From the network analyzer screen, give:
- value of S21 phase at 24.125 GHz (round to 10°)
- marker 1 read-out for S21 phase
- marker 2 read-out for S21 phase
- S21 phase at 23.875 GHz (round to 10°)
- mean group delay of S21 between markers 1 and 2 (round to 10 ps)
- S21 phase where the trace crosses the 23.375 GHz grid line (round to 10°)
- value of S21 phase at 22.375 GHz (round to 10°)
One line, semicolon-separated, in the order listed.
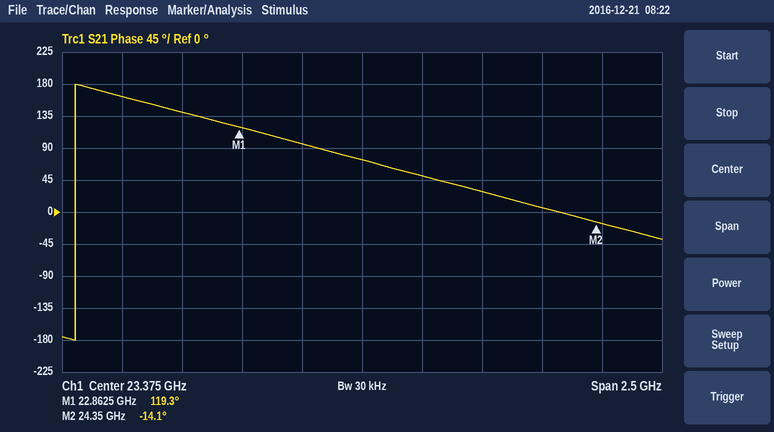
10°; 119.3°; -14.1°; 30°; 250 ps; 70°; 160°
